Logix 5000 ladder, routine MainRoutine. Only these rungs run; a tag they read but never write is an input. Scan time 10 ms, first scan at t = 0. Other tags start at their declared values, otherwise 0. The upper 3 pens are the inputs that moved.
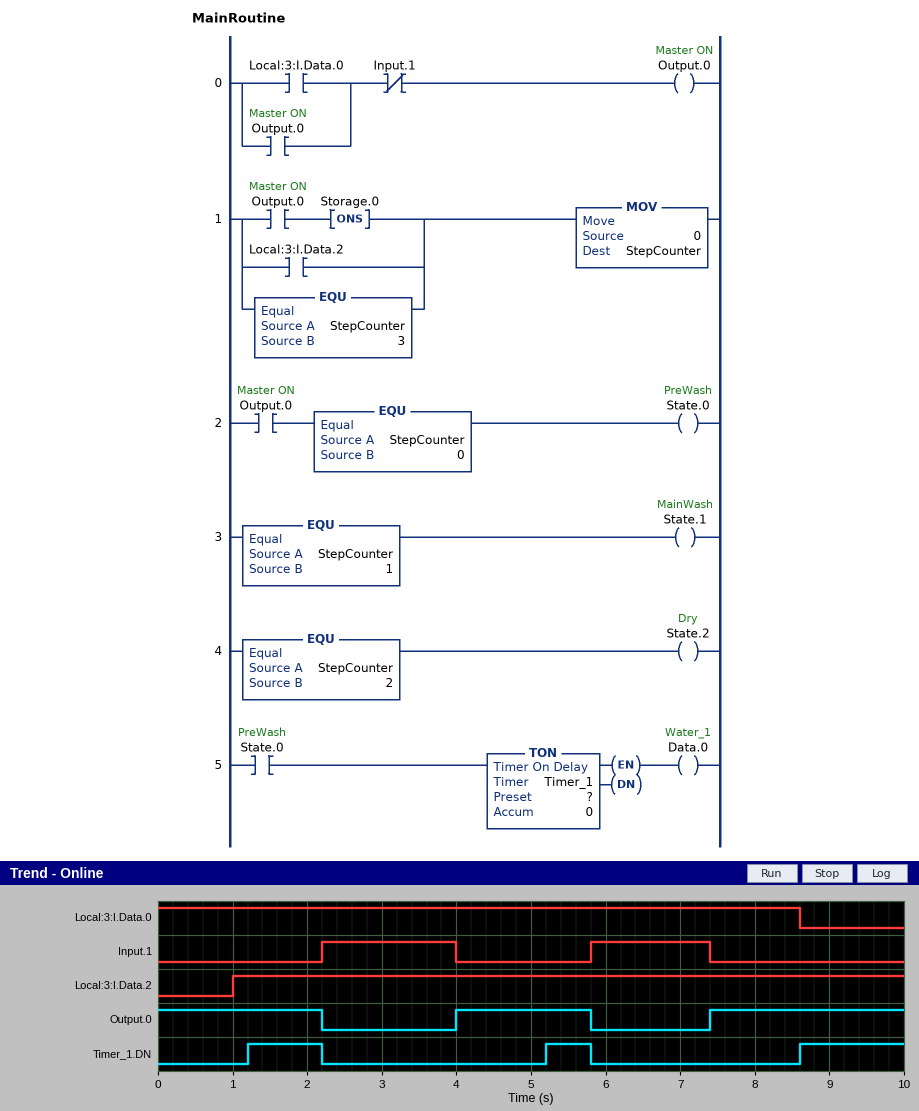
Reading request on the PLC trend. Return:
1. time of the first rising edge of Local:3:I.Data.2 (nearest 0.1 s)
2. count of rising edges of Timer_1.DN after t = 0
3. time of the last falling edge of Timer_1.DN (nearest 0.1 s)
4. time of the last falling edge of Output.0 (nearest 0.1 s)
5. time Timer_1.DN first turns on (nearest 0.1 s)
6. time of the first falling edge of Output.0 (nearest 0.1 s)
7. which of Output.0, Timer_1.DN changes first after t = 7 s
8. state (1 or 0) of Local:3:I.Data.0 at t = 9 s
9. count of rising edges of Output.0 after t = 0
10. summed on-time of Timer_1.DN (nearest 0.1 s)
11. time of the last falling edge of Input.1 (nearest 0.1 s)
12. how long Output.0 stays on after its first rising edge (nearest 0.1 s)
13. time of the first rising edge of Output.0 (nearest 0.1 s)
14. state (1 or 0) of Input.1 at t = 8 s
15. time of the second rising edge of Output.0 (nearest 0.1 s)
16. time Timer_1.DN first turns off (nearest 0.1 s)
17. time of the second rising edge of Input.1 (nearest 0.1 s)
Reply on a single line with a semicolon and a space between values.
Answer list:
1.0 s; 3; 5.8 s; 5.8 s; 1.2 s; 2.2 s; Output.0; 0; 2; 3.0 s; 7.4 s; 1.8 s; 4.0 s; 0; 7.4 s; 2.2 s; 5.8 s
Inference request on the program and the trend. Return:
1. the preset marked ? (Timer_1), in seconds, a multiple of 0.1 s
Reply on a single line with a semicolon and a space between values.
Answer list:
1.2 s
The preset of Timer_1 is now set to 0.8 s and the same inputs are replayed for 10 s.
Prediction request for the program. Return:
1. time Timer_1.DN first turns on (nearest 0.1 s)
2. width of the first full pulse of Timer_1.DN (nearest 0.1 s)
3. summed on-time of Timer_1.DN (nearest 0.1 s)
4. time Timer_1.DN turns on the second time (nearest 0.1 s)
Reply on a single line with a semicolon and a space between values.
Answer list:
0.8 s; 1.4 s; 4.2 s; 4.8 s
